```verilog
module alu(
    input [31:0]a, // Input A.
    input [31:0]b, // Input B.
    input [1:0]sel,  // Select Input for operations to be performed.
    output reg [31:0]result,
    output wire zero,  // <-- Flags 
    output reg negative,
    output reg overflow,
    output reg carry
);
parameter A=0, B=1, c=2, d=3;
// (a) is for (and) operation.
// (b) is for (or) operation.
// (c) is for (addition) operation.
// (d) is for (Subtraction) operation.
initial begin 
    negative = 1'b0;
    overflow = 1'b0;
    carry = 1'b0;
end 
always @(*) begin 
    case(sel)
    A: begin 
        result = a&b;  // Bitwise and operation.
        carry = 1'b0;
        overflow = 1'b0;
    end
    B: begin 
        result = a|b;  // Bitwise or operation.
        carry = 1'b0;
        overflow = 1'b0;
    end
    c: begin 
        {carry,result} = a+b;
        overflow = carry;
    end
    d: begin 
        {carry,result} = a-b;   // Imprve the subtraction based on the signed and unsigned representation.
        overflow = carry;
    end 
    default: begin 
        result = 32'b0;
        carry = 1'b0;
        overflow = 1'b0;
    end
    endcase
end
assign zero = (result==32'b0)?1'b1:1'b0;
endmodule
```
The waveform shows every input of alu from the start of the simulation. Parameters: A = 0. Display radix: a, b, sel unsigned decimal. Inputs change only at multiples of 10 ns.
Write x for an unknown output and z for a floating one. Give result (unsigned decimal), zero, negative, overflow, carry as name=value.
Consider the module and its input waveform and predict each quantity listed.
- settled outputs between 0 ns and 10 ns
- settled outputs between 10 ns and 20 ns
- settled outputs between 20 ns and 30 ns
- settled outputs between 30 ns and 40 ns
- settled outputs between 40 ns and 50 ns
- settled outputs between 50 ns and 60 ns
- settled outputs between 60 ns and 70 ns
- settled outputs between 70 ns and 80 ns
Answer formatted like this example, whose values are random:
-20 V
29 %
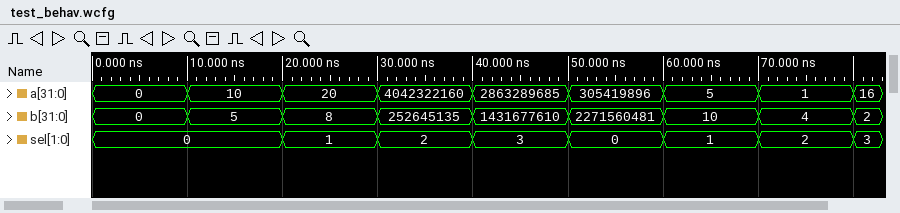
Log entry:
result=0, zero=1, negative=0, overflow=0, carry=0
result=0, zero=1, negative=0, overflow=0, carry=0
result=28, zero=0, negative=0, overflow=0, carry=0
result=4294967295, zero=0, negative=0, overflow=0, carry=0
result=1431612075, zero=0, negative=0, overflow=0, carry=0
result=35930656, zero=0, negative=0, overflow=0, carry=0
result=15, zero=0, negative=0, overflow=0, carry=0
result=5, zero=0, negative=0, overflow=0, carry=0
